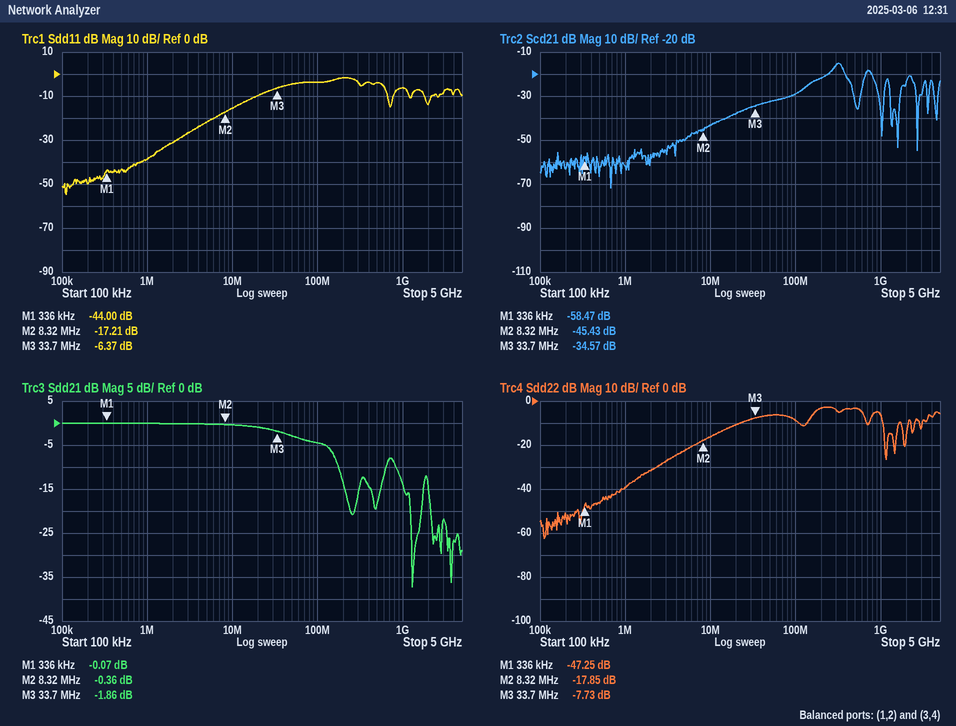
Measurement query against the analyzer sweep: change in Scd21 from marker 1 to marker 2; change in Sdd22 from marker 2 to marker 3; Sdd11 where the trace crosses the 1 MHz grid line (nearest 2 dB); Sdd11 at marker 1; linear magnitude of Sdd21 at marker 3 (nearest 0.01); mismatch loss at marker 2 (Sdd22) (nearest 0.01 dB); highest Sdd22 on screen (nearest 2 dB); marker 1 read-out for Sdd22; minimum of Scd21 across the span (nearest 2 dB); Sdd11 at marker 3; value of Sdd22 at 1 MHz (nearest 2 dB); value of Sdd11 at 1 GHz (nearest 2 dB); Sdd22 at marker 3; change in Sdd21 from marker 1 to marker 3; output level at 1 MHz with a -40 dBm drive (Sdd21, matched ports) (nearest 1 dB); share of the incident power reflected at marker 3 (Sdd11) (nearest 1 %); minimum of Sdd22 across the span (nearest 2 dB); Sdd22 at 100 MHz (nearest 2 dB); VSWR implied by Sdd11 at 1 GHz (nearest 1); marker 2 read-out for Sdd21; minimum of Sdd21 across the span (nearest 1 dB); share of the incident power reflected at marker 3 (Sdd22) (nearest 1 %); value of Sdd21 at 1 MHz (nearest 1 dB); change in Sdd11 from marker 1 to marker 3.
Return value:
13.04 dB
10.12 dB
-38 dB
-44.00 dB
0.81
0.07 dB
-2 dB
-47.25 dB
-72 dB
-6.37 dB
-40 dB
-6 dB
-7.73 dB
-1.79 dB
-40 dBm
23 %
-62 dB
-8 dB
3
-0.36 dB
-37 dB
17 %
0 dB
37.63 dB
